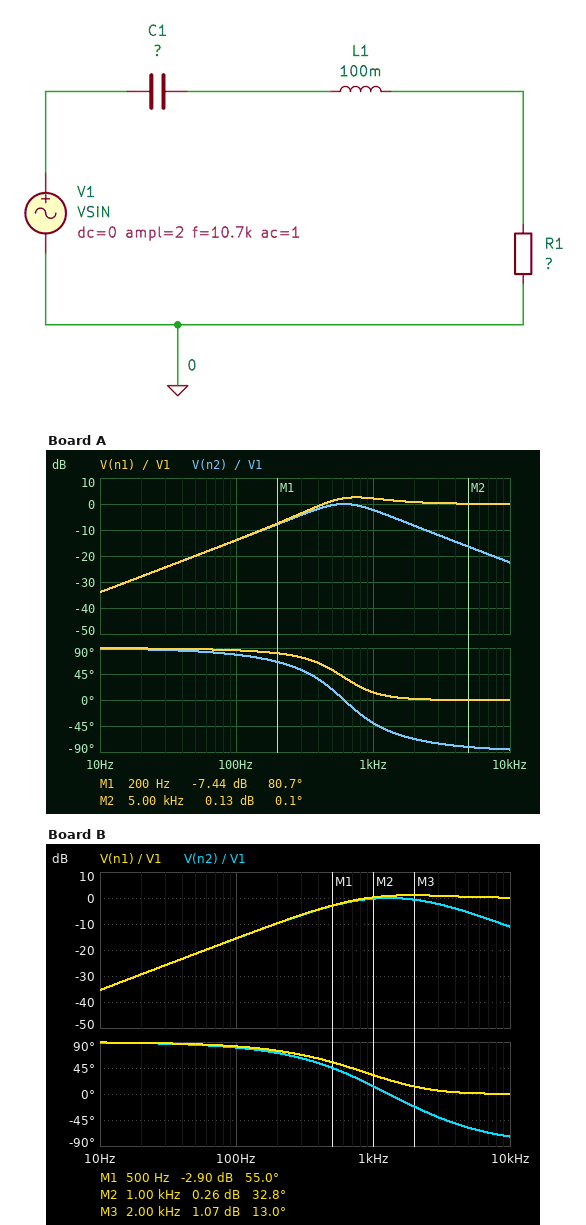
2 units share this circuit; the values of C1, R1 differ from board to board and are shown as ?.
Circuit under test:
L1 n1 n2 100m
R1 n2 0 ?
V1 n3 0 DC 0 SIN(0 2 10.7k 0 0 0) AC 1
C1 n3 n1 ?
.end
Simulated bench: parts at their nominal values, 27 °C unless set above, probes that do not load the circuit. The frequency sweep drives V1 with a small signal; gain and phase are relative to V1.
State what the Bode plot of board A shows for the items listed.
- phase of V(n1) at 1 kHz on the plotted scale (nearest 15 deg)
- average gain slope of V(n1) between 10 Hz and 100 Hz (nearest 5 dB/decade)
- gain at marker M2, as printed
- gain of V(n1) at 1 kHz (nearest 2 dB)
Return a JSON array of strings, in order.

["15 deg", "20 dB/decade", "0.13 dB", "2 dB"]
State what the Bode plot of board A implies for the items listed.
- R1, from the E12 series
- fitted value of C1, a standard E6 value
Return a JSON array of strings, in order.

["470 Ω", "680 nF"]
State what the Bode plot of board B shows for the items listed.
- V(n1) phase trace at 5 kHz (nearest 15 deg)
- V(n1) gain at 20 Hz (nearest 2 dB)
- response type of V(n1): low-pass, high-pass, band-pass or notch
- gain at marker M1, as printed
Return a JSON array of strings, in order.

["0 deg", "-30 dB", "high-pass", "-2.90 dB"]
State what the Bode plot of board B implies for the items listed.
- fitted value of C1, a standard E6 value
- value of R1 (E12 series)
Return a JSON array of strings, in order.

["150 nF", "1.8 kΩ"]
